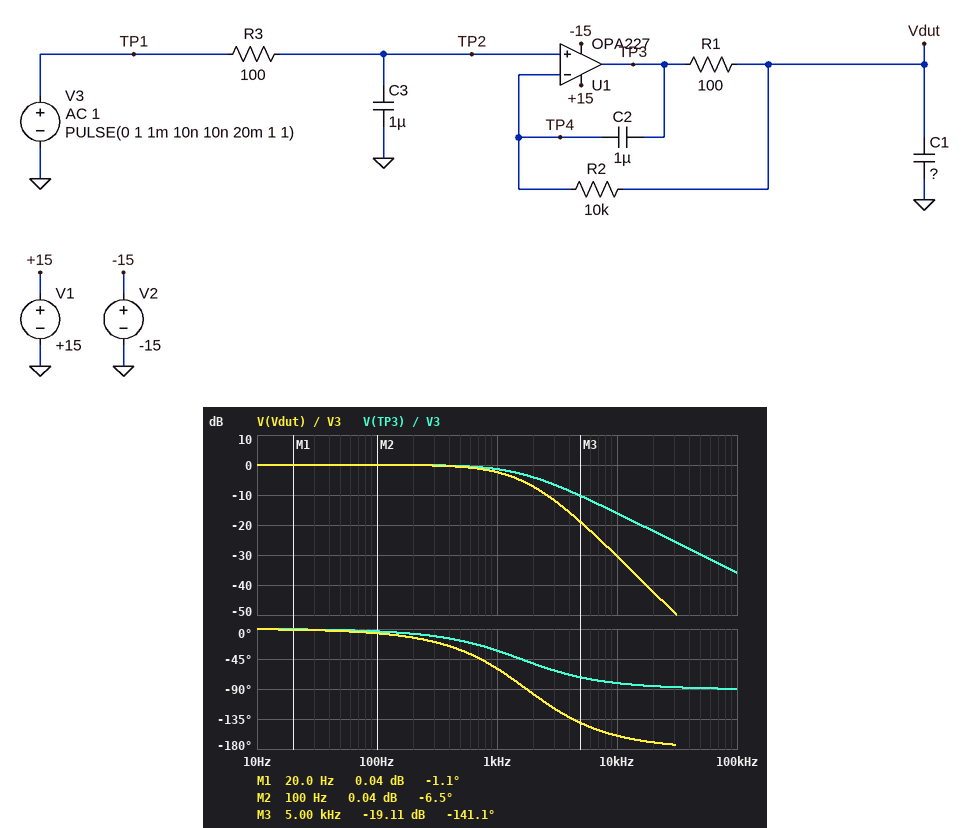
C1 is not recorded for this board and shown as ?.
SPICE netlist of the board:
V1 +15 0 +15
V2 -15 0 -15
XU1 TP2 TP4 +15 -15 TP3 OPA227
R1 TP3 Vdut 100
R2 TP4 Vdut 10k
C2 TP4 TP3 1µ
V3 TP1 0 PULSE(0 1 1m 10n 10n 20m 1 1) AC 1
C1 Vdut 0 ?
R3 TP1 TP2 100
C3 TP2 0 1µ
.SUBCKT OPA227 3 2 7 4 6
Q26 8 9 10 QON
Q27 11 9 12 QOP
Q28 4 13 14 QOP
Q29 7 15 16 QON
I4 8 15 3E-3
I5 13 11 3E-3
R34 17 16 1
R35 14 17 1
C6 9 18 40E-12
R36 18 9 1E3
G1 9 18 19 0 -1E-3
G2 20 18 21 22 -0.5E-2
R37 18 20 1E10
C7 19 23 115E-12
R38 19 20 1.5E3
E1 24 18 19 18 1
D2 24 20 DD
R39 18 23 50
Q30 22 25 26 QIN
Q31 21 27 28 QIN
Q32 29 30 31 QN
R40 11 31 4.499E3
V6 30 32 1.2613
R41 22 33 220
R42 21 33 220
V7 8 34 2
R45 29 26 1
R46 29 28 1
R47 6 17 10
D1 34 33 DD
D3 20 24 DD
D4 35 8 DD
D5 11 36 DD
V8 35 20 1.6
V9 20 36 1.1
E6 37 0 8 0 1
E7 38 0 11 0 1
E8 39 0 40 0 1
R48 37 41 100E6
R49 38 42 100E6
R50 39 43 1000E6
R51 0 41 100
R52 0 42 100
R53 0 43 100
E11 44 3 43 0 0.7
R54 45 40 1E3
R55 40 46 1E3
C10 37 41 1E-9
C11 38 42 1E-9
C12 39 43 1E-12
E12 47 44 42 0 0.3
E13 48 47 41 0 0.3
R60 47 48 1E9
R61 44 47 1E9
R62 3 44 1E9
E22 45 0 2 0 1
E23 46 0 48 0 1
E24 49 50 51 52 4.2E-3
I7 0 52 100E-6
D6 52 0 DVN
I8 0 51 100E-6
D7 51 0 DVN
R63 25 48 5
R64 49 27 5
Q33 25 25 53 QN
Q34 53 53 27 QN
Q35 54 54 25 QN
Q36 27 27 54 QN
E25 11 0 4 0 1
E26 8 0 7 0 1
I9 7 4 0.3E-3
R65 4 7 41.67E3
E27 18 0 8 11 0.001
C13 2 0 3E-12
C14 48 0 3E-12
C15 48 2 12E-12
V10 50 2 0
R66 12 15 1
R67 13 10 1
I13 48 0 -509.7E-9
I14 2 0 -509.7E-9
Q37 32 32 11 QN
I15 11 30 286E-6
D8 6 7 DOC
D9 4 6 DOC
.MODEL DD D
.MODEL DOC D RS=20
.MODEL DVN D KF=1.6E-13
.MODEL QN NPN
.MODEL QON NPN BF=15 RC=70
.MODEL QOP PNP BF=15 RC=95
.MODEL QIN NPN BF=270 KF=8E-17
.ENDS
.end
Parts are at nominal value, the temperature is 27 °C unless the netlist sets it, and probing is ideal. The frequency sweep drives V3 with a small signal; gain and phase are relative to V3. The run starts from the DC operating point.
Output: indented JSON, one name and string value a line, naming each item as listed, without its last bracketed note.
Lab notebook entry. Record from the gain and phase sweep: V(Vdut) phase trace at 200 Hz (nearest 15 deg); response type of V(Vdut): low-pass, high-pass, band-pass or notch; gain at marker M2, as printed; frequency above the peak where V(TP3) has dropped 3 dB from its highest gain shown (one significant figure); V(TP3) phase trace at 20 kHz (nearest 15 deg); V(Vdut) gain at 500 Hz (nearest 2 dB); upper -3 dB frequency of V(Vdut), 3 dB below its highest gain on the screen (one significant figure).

{
  "V(Vdut) phase trace at 200 Hz": "-15 deg",
  "response type of V(Vdut): low-pass, high-pass, band-pass or notch": "low-pass",
  "gain at marker M2, as printed": "0.04 dB",
  "frequency above the peak where V(TP3) has dropped 3 dB from its highest gain shown": "2 kHz",
  "V(TP3) phase trace at 20 kHz": "-90 deg",
  "V(Vdut) gain at 500 Hz": "0 dB",
  "upper -3 dB frequency of V(Vdut), 3 dB below its highest gain on the screen": "1 kHz"
}
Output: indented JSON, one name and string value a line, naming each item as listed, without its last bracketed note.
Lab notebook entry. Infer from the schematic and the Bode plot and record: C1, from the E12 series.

{
  "C1, from the E12 series": "820 nF"
}
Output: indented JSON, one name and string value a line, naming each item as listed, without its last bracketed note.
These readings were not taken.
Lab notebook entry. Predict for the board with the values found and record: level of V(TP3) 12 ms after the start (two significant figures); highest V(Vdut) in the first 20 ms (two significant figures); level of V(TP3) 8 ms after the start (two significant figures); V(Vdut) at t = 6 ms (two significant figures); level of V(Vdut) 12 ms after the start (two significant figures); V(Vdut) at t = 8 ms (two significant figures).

{
  "level of V(TP3) 12 ms after the start": "1.0 V",
  "highest V(Vdut) in the first 20 ms": "1.0 V",
  "level of V(TP3) 8 ms after the start": "1.0 V",
  "V(Vdut) at t = 6 ms": "1.0 V",
  "level of V(Vdut) 12 ms after the start": "1.0 V",
  "V(Vdut) at t = 8 ms": "1.0 V"
}
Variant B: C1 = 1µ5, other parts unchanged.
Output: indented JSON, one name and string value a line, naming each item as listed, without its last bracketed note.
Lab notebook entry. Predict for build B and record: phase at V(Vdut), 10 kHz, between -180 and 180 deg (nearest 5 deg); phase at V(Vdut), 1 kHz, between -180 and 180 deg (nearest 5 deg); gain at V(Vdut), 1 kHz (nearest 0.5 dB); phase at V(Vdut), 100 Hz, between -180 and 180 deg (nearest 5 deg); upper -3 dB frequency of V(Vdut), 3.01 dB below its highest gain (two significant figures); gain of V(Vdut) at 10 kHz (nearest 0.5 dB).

{
  "phase at V(Vdut), 10 kHz, between -180 and 180 deg": "-165 deg",
  "phase at V(Vdut), 1 kHz, between -180 and 180 deg": "-75 deg",
  "gain at V(Vdut), 1 kHz": "-4.0 dB",
  "phase at V(Vdut), 100 Hz, between -180 and 180 deg": "-10 deg",
  "upper -3 dB frequency of V(Vdut), 3.01 dB below its highest gain": "810 Hz",
  "gain of V(Vdut) at 10 kHz": "-35.5 dB"
}
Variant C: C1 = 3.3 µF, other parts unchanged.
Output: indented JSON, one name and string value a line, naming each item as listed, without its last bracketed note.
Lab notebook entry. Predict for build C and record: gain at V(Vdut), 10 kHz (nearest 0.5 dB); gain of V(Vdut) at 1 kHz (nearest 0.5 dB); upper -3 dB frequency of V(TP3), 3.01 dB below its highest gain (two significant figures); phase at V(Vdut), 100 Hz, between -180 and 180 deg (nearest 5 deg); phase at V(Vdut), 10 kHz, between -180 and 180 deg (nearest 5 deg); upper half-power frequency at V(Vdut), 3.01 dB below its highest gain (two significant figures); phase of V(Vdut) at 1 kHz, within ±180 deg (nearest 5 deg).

{
  "gain at V(Vdut), 10 kHz": "-42.5 dB",
  "gain of V(Vdut) at 1 kHz": "-8.5 dB",
  "upper -3 dB frequency of V(TP3), 3.01 dB below its highest gain": "1.5 kHz",
  "phase at V(Vdut), 100 Hz, between -180 and 180 deg": "-15 deg",
  "phase at V(Vdut), 10 kHz, between -180 and 180 deg": "-170 deg",
  "upper half-power frequency at V(Vdut), 3.01 dB below its highest gain": "440 Hz",
  "phase of V(Vdut) at 1 kHz, within ±180 deg": "-95 deg"
}
